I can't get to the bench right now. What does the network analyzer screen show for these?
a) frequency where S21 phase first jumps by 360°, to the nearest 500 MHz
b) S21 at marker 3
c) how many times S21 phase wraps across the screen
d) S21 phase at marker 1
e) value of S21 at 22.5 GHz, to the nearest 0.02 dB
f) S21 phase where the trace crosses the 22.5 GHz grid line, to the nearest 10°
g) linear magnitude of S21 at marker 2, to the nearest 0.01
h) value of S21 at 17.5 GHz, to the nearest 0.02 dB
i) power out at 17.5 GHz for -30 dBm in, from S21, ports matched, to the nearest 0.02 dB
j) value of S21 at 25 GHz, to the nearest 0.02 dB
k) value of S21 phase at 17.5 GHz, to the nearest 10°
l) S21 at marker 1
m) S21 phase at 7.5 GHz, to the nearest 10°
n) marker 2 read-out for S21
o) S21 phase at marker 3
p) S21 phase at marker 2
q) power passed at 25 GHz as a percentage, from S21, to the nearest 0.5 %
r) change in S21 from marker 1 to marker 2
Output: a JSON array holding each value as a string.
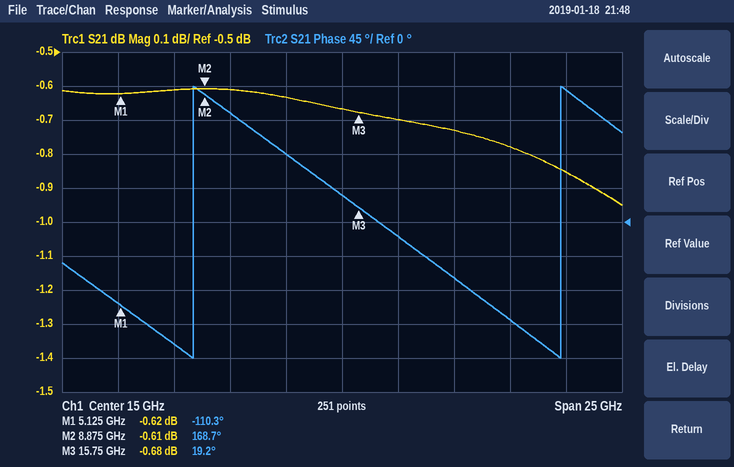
["8.5 GHz", "-0.68 dB", "2", "-110.3°", "-0.78 dB", "-130°", "0.93", "-0.70 dB", "-30.70 dBm", "-0.86 dB", "-20°", "-0.62 dB", "-160°", "-0.61 dB", "19.2°", "168.7°", "82.0 %", "0.01 dB"]
